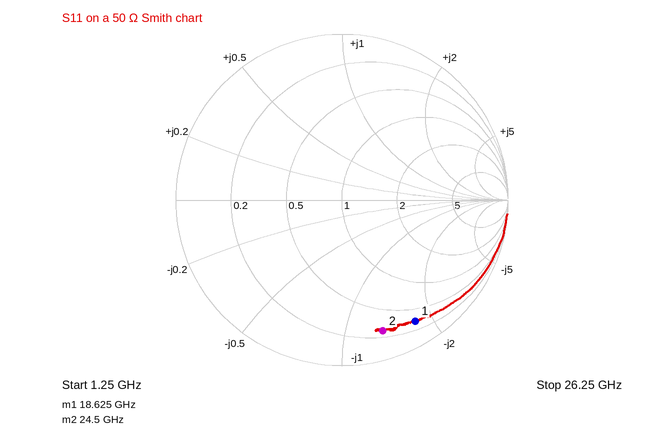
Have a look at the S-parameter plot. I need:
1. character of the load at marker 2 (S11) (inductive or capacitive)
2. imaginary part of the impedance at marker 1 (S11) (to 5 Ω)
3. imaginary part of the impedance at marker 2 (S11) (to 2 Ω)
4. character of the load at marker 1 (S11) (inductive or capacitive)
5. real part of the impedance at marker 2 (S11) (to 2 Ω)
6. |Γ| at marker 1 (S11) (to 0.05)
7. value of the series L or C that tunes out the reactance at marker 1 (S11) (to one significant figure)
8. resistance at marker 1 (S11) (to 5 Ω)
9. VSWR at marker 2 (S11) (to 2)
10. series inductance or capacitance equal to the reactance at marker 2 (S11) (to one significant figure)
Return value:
capacitive
-85 Ω
-66 Ω
capacitive
14 Ω
0.85
700 pH
15 Ω
10
100 fF
